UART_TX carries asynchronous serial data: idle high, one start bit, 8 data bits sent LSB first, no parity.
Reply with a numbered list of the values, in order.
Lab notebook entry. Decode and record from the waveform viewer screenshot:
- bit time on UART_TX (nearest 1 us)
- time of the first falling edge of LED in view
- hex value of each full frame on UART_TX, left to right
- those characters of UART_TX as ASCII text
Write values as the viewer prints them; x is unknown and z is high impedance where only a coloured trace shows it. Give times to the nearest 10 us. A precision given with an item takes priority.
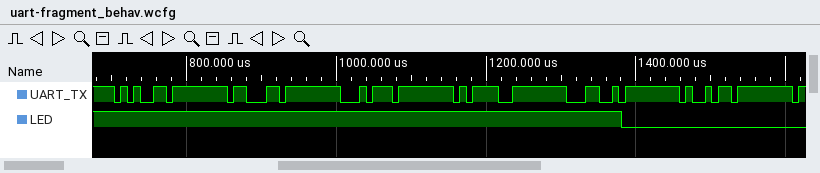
1. 9 us
2. 1380 us
3. 65, 63, 74, 3D, 4C, 69
4. "ect=Li"
